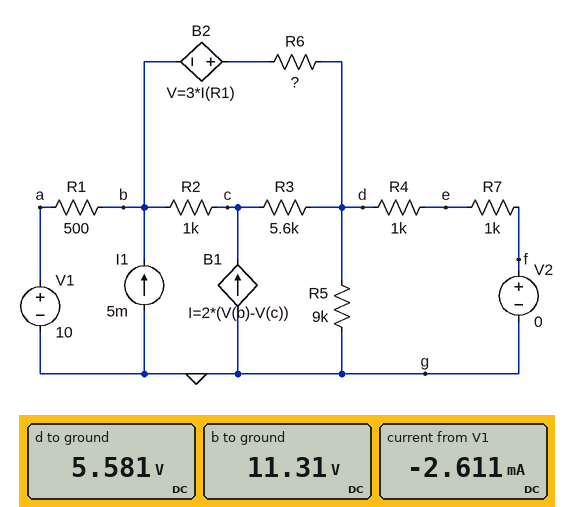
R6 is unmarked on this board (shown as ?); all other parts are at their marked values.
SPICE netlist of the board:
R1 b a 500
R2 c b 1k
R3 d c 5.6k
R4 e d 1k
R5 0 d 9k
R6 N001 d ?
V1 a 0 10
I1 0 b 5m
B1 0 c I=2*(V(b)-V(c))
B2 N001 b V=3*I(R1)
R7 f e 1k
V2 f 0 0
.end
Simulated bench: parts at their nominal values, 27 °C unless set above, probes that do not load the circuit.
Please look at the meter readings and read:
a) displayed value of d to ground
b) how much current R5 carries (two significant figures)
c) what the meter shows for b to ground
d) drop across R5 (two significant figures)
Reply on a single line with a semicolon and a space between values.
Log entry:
5.581 V; 620 µA; 11.31 V; 5.6 V
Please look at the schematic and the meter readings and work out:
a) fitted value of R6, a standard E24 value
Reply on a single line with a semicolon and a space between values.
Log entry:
2.4 kΩ
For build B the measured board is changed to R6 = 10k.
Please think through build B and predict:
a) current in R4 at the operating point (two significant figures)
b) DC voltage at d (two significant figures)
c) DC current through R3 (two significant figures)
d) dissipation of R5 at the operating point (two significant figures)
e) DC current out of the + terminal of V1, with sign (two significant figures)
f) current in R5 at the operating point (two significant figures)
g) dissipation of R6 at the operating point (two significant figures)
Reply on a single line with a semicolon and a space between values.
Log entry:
1.9 mA; 3.8 V; 1.5 mA; 1.6 mW; -4.2 mA; 420 µA; 6.9 mW
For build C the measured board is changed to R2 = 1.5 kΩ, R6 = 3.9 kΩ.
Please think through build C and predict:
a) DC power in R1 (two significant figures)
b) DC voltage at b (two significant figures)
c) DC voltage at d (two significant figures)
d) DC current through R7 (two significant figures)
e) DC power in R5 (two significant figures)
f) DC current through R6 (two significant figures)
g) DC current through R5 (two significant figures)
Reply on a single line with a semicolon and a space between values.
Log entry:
5.3 mW; 12 V; 4.8 V; 2.4 mA; 2.6 mW; 1.7 mA; 540 µA
